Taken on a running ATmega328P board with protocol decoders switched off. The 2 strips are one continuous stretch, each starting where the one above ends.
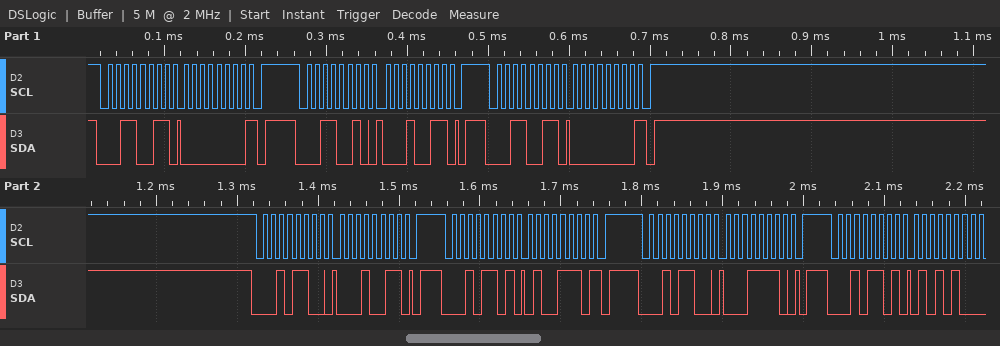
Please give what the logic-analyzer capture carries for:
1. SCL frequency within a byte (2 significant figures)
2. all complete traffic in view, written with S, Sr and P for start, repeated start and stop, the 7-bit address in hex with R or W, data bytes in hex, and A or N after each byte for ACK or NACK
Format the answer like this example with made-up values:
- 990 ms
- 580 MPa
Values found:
- 100 kHz
- S 19R A 00 N P S 19W A 13 A P S 19R A 00 N P S 16W A 13 A P S 16R A 4E N P S 16W A 1E A P S 16R A 54 A
